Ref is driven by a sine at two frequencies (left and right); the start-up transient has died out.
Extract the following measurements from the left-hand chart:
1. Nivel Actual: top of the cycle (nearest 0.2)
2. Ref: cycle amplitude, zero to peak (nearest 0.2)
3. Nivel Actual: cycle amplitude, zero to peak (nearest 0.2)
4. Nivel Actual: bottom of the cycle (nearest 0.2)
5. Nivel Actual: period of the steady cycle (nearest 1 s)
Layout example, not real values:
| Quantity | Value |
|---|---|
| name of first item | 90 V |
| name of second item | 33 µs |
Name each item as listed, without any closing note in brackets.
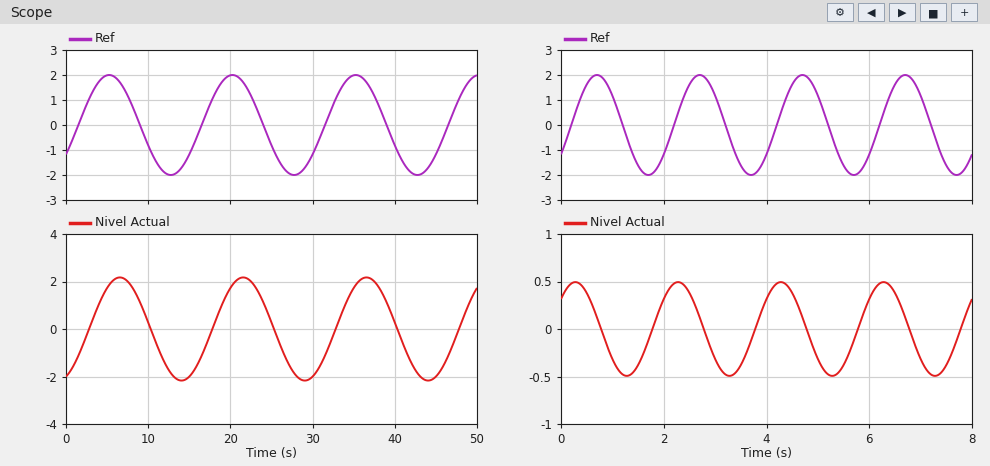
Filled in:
| Quantity | Value |
|---|---|
| Nivel Actual: top of the cycle | 2.2 |
| Ref: cycle amplitude, zero to peak | 2.0 |
| Nivel Actual: cycle amplitude, zero to peak | 2.2 |
| Nivel Actual: bottom of the cycle | -2.2 |
| Nivel Actual: period of the steady cycle | 15 s |
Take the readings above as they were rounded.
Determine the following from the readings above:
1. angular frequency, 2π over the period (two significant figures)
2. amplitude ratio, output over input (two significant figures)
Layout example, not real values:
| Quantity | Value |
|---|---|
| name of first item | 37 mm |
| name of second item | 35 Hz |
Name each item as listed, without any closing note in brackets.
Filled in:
| Quantity | Value |
|---|---|
| angular frequency, 2π over the period | 0.42 rad/s |
| amplitude ratio, output over input | 1.1 |
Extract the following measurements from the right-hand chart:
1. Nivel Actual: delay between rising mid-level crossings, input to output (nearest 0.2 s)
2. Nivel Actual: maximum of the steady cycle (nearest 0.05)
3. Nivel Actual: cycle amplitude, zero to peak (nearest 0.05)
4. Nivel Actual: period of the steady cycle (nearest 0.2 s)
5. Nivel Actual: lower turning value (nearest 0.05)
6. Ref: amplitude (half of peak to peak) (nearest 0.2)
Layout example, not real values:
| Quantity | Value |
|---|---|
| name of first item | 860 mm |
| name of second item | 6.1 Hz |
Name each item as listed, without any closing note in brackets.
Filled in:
| Quantity | Value |
|---|---|
| Nivel Actual: delay between rising mid-level crossings, input to output | 1.6 s |
| Nivel Actual: maximum of the steady cycle | 0.50 |
| Nivel Actual: cycle amplitude, zero to peak | 0.50 |
| Nivel Actual: period of the steady cycle | 2.0 s |
| Nivel Actual: lower turning value | -0.50 |
| Ref: amplitude (half of peak to peak) | 2.0 |
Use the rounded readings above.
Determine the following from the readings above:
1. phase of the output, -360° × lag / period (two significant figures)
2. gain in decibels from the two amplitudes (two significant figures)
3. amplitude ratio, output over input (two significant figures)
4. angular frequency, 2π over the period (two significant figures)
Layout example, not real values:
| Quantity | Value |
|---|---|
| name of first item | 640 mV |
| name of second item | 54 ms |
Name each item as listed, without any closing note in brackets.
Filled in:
| Quantity | Value |
|---|---|
| phase of the output, -360° × lag / period | -290° |
| gain in decibels from the two amplitudes | -12 dB |
| amplitude ratio, output over input | 0.25 |
| angular frequency, 2π over the period | 3.1 rad/s |
